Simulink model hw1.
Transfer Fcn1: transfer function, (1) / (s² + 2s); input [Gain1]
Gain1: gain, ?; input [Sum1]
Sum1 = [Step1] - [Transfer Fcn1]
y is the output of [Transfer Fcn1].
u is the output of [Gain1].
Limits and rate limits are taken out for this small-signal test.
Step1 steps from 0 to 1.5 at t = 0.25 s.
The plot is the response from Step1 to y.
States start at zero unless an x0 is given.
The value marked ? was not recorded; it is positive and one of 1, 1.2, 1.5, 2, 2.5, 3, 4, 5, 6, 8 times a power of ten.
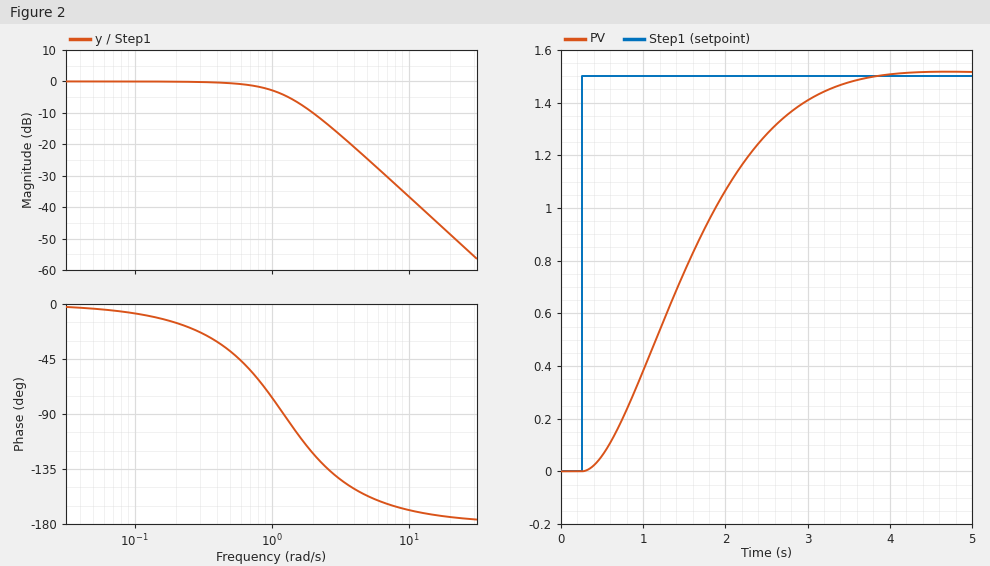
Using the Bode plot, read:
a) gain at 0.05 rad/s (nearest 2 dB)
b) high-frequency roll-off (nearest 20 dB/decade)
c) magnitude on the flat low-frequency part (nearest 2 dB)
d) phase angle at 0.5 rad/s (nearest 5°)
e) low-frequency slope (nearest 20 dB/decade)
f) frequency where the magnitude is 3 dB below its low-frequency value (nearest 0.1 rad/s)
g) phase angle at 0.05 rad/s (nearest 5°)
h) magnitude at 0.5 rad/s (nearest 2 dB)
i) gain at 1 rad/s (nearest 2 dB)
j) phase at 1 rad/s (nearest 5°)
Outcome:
0 dB
-40 dB/decade
0 dB
-40°
0 dB/decade
1.0 rad/s
-5°
0 dB
-2 dB
-75°
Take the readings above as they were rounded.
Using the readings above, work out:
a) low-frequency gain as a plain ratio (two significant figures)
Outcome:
1.0
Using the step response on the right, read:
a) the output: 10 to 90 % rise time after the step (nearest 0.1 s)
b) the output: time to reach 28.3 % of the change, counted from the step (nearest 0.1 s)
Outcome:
2.1 s
0.8 s
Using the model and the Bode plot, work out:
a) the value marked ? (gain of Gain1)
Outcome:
1.5
